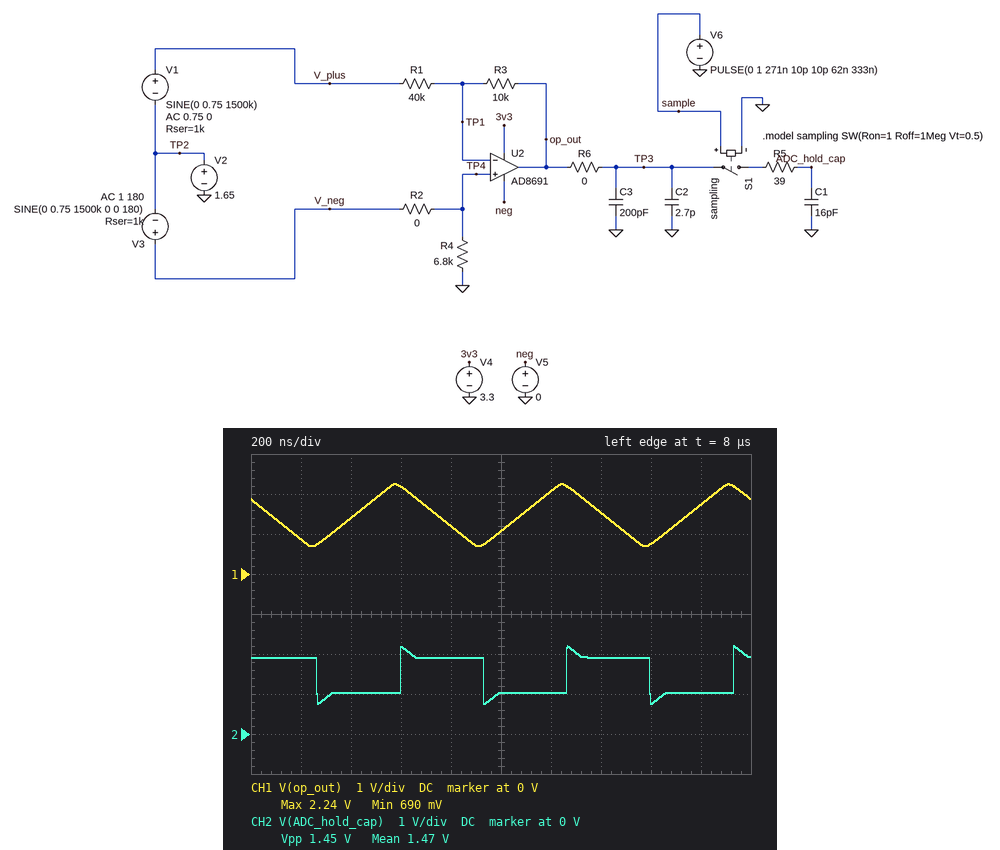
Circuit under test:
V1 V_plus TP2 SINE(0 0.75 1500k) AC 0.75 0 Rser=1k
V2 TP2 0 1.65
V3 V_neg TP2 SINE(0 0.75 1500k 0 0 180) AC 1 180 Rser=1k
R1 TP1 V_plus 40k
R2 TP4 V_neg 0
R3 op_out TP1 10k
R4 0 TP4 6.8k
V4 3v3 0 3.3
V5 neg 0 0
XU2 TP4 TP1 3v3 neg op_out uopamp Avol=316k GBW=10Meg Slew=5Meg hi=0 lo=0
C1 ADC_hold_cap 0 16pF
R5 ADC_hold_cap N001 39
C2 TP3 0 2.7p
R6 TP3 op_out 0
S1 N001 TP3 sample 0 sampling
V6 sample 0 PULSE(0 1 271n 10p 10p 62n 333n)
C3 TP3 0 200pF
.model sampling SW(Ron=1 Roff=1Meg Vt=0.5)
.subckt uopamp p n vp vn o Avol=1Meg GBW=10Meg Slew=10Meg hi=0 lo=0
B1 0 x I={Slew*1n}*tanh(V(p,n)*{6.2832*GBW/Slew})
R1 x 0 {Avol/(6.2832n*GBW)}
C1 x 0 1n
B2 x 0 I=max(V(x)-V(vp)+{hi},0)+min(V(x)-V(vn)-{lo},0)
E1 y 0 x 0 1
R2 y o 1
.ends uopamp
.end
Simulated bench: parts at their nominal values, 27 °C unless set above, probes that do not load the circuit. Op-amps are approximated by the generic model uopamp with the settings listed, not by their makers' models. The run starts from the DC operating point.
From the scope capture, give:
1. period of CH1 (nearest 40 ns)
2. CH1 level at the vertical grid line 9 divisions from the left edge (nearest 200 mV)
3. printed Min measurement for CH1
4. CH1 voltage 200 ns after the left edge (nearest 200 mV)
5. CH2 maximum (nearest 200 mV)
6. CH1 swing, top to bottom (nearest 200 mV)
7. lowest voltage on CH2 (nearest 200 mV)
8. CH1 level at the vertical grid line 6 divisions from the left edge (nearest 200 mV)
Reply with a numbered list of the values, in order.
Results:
1. 680 ns
2. 1.8 V
3. 690 mV
4. 800 mV
5. 2.2 V
6. 1.6 V
7. 800 mV
8. 2.0 V
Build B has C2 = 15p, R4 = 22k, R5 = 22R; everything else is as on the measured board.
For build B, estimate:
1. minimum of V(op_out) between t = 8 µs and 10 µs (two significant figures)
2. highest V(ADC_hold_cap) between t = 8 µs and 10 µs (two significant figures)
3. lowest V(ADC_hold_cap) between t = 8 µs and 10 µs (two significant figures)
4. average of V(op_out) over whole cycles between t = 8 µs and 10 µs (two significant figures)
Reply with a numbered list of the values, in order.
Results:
1. 910 mV
2. 2.5 V
3. 930 mV
4. 1.7 V
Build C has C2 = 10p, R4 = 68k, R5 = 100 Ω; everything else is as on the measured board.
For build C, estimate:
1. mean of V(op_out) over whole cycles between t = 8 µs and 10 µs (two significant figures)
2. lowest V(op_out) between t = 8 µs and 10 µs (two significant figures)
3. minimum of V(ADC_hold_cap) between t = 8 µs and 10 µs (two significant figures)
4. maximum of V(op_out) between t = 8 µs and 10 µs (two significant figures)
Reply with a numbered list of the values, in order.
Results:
1. 1.7 V
2. 910 mV
3. 950 mV
4. 2.5 V
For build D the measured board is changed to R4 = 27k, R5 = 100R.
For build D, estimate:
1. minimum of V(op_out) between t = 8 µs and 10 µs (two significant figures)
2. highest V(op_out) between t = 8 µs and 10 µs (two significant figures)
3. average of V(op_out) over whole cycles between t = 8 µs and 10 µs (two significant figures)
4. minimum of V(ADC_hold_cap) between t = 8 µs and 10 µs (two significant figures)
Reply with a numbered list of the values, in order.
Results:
1. 910 mV
2. 2.5 V
3. 1.7 V
4. 950 mV
